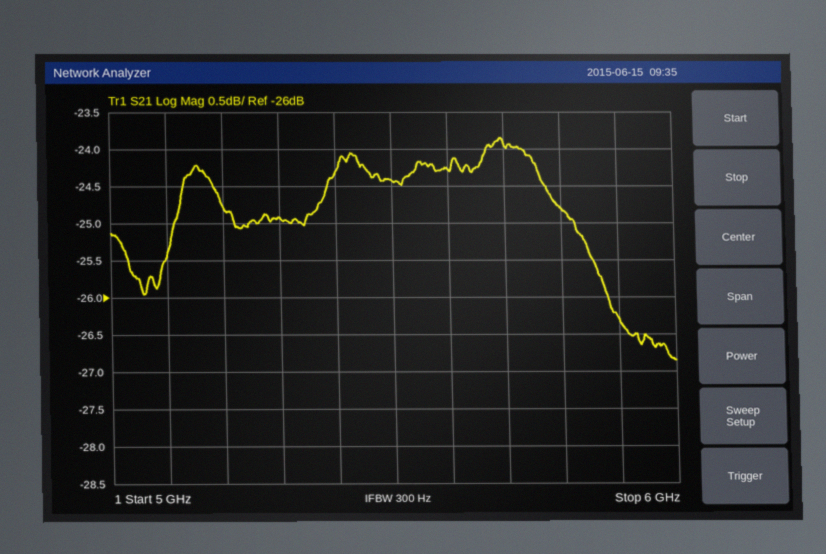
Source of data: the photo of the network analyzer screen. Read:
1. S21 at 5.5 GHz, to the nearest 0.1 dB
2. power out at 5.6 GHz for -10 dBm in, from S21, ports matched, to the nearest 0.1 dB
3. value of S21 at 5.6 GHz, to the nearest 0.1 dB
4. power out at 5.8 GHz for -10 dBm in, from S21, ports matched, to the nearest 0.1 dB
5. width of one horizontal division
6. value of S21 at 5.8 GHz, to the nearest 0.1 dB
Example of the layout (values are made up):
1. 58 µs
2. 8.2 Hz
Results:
1. -24.4 dB
2. -34.3 dBm
3. -24.3 dB
4. -34.8 dBm
5. 100 MHz
6. -24.8 dB
